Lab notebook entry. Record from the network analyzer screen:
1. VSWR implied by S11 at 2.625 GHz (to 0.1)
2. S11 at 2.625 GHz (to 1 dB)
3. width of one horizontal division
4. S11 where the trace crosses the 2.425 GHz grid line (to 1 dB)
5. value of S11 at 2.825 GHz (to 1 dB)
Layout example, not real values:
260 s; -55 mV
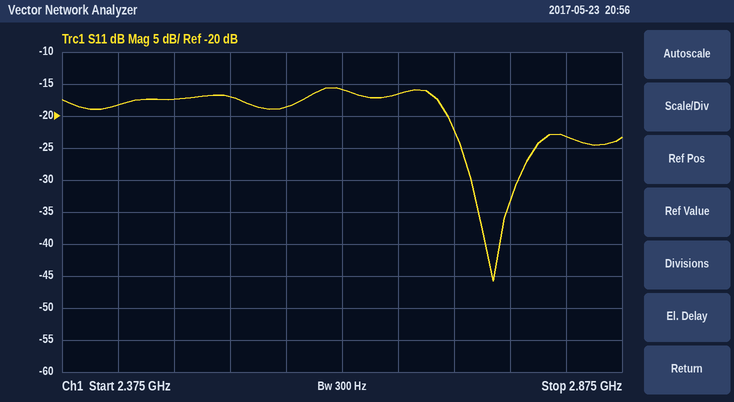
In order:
1.4; -16 dB; 50 MHz; -18 dB; -23 dB
